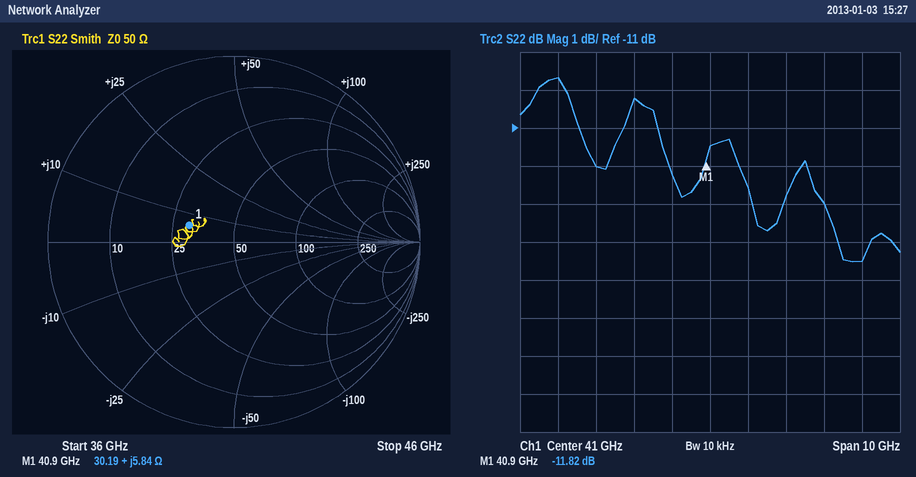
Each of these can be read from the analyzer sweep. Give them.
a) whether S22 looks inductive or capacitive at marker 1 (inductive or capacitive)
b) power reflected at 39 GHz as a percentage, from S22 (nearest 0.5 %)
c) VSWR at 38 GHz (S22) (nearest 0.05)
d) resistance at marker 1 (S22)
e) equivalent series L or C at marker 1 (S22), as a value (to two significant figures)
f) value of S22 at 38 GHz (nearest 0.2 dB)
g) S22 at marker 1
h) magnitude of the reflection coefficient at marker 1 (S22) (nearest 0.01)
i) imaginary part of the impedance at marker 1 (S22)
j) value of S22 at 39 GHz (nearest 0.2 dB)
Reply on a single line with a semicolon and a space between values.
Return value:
inductive; 9.5 %; 1.65; 30.19 Ω; 23 pH; -12.0 dB; -11.82 dB; 0.26; +5.84 Ω; -10.2 dB
